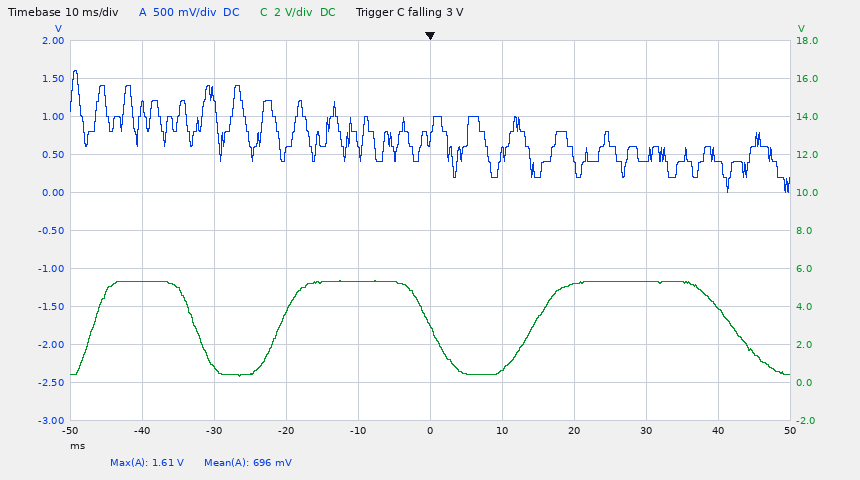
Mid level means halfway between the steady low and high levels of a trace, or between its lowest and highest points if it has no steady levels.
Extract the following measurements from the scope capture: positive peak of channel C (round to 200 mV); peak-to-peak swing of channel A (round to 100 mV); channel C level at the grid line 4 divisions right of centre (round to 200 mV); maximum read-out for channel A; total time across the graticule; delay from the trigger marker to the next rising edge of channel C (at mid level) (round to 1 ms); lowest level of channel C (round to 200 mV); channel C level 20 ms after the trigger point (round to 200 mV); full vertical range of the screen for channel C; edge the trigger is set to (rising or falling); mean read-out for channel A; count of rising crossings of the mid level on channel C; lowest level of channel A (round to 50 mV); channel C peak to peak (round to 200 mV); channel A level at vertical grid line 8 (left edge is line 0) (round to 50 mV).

5.4 V
1.60 V
4.0 V
1.61 V
100 ms
14 ms
400 mV
5.2 V
20 V
falling
696 mV
3
0 mV
5.0 V
450 mV
